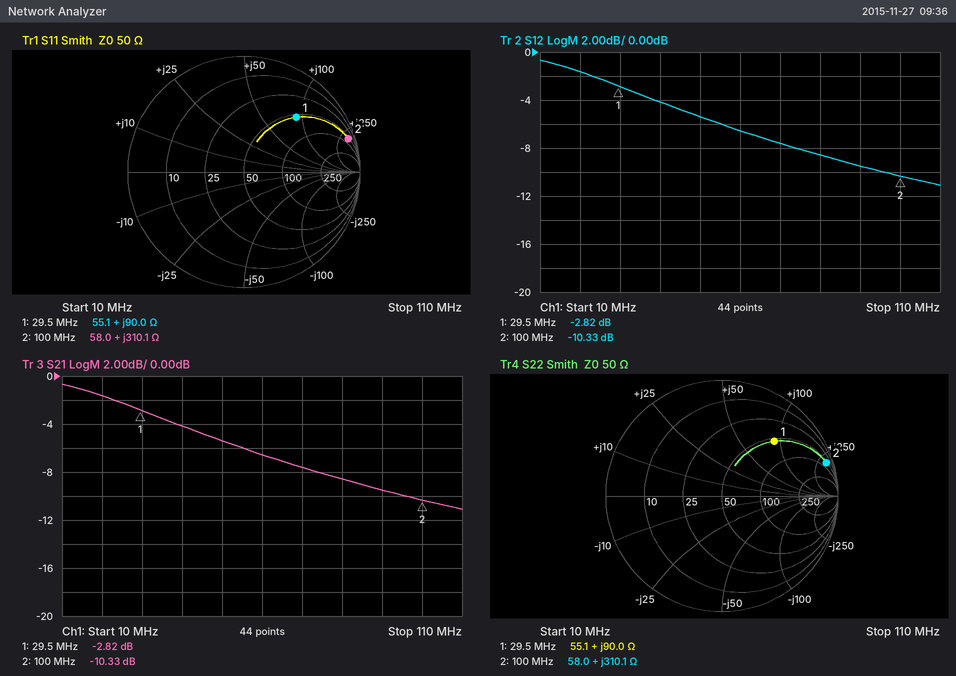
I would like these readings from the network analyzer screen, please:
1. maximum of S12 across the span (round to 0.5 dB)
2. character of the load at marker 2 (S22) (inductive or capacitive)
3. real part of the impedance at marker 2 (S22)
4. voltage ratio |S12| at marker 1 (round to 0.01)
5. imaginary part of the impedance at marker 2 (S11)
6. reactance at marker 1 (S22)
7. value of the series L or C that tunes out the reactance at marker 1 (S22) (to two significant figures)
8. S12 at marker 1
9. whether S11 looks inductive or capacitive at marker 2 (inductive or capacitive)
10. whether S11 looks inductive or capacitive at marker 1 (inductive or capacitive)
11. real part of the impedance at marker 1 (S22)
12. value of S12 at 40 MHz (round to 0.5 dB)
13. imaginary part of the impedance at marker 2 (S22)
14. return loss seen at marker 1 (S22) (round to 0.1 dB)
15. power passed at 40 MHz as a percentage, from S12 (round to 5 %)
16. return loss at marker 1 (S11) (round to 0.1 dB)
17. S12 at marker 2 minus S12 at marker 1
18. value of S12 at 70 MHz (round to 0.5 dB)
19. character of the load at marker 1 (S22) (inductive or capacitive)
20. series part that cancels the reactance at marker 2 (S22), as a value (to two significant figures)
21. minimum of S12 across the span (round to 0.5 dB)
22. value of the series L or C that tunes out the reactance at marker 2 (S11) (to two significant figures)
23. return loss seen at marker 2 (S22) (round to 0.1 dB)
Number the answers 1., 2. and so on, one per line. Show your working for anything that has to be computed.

1. -0.5 dB
2. inductive
3. 58.0 Ω
4. 10^(-2.82/20) ≈ 0.72
5. +310.1 Ω
6. +90.0 Ω
7. C = 1/(2π × 29.5 MHz × 90 Ω) ≈ 60 pF
8. -2.82 dB
9. inductive
10. inductive
11. 55.1 Ω
12. -4.0 dB
13. +310.1 Ω
14. 3.7 dB
15. 10^(-4/10) ≈ 40 %
16. 3.7 dB
17. -10.33 − (-2.82) = -7.51 dB
18. -7.5 dB
19. inductive
20. C = 1/(2π × 100 MHz × 310.1 Ω) ≈ 5.1 pF
21. -11.0 dB
22. C = 1/(2π × 100 MHz × 310.1 Ω) ≈ 5.1 pF
23. 0.5 dB
